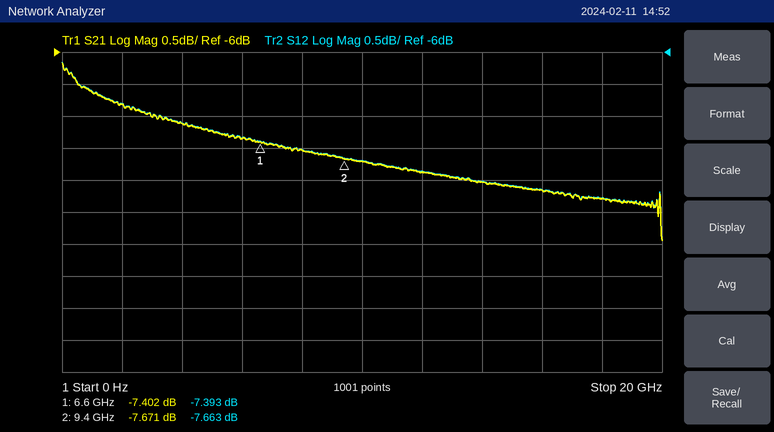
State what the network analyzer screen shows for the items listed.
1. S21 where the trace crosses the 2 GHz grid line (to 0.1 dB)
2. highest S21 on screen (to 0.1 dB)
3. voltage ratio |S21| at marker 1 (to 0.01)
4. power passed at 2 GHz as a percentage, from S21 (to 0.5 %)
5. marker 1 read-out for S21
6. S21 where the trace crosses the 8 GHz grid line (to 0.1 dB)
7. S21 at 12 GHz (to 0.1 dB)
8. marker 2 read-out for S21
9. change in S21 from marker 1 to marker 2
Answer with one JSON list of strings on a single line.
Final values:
["-6.8 dB", "-6.2 dB", "0.43", "21.0 %", "-7.402 dB", "-7.5 dB", "-7.9 dB", "-7.671 dB", "-0.269 dB"]
